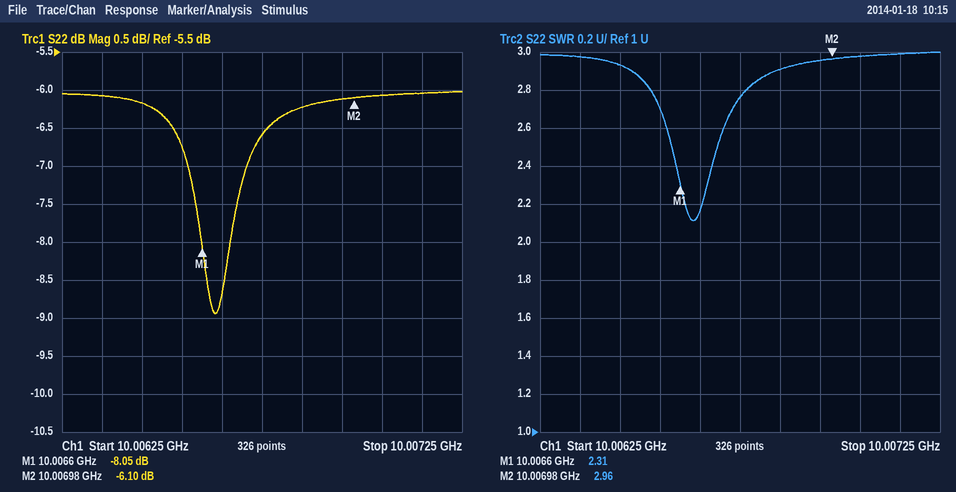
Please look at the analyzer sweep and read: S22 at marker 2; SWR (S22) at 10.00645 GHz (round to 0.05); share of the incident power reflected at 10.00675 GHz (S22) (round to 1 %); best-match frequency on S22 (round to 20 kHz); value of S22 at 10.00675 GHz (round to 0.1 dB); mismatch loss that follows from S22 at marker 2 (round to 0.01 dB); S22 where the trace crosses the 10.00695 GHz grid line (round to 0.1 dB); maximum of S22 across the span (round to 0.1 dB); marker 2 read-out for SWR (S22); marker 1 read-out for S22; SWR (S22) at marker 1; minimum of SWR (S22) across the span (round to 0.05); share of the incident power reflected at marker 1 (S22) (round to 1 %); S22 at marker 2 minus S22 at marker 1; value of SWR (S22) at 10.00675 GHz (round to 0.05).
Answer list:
-6.10 dB
2.95
22 %
10.00664 GHz
-6.6 dB
1.22 dB
-6.1 dB
-6.0 dB
2.96
-8.05 dB
2.31
2.10
16 %
1.95 dB
2.75
